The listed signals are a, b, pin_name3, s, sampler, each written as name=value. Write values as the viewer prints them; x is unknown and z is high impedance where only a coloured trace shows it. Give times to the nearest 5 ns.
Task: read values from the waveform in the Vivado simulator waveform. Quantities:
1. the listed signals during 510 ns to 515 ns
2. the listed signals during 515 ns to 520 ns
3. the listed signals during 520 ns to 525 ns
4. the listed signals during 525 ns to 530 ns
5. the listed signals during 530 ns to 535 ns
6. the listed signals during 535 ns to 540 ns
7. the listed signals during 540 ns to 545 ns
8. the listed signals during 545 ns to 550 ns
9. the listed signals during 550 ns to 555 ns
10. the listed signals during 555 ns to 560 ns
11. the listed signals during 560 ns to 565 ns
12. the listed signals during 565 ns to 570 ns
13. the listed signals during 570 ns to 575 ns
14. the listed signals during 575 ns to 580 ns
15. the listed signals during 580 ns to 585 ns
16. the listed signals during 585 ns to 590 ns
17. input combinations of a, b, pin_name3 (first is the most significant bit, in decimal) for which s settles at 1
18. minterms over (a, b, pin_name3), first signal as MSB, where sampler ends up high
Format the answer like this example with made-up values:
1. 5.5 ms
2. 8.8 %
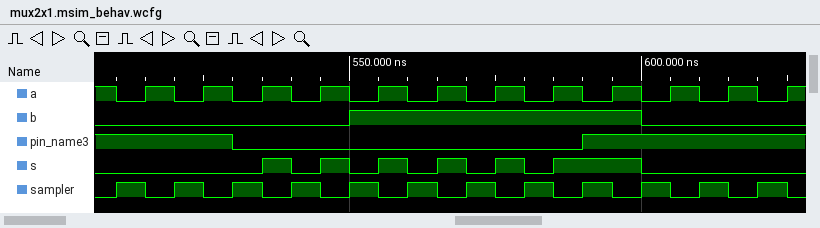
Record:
1. a=0, b=0, pin_name3=1, s=0, sampler=1
2. a=1, b=0, pin_name3=1, s=0, sampler=0
3. a=0, b=0, pin_name3=1, s=0, sampler=1
4. a=1, b=0, pin_name3=1, s=0, sampler=0
5. a=0, b=0, pin_name3=0, s=0, sampler=1
6. a=1, b=0, pin_name3=0, s=1, sampler=0
7. a=0, b=0, pin_name3=0, s=0, sampler=1
8. a=1, b=0, pin_name3=0, s=1, sampler=0
9. a=0, b=1, pin_name3=0, s=0, sampler=1
10. a=1, b=1, pin_name3=0, s=1, sampler=0
11. a=0, b=1, pin_name3=0, s=0, sampler=1
12. a=1, b=1, pin_name3=0, s=1, sampler=0
13. a=0, b=1, pin_name3=0, s=0, sampler=1
14. a=1, b=1, pin_name3=0, s=1, sampler=0
15. a=0, b=1, pin_name3=0, s=0, sampler=1
16. a=1, b=1, pin_name3=0, s=1, sampler=0
17. 3, 4, 6, 7
18. 0, 1, 2, 3
